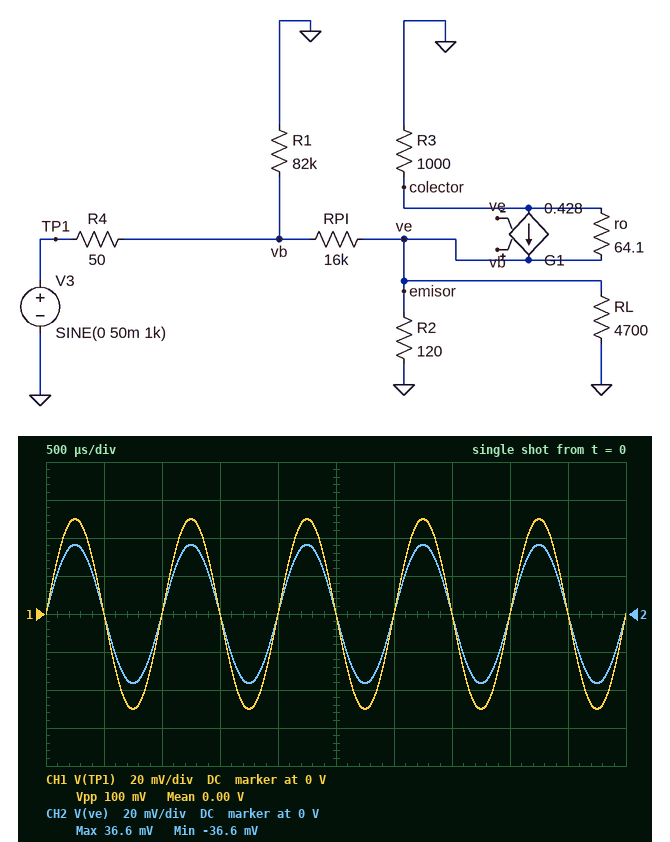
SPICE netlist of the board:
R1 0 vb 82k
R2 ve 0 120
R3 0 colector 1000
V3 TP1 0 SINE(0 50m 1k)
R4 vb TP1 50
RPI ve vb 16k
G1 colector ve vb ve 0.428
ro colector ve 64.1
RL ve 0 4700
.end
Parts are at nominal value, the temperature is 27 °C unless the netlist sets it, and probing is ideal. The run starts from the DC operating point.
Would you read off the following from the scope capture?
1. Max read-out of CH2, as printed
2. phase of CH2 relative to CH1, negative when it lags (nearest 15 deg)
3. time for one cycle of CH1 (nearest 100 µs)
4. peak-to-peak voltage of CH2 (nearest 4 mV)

36.6 mV
0 deg
1.0 ms
72 mV
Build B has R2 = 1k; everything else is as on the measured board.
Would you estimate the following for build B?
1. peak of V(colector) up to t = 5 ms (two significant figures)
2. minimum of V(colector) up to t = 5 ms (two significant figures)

56 mV
-56 mV
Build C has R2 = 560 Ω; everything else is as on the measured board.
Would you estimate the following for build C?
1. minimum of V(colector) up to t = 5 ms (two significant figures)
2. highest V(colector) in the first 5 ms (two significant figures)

-89 mV
89 mV
